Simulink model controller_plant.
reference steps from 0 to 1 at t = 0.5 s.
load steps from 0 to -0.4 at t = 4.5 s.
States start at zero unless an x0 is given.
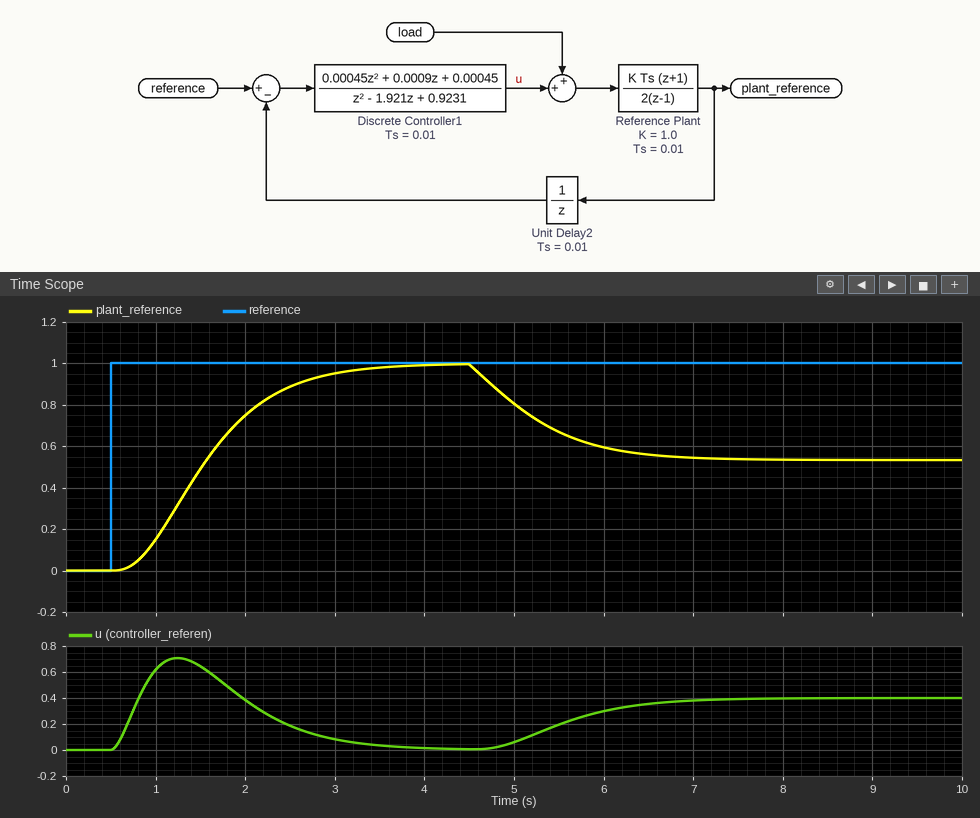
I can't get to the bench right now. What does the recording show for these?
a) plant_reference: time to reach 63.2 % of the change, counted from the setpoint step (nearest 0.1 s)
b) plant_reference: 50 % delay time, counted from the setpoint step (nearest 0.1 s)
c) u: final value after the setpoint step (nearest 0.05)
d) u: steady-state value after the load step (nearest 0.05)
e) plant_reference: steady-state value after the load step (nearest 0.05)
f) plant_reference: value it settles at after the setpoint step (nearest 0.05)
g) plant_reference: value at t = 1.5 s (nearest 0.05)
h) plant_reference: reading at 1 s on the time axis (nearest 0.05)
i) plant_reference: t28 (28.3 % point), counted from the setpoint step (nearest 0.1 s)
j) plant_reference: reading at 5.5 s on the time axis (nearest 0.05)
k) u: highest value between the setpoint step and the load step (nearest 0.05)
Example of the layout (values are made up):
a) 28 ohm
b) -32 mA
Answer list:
a) 1.2 s
b) 1.0 s
c) 0.00
d) 0.40
e) 0.55
f) 1.00
g) 0.50
h) 0.15
i) 0.7 s
j) 0.65
k) 0.70
